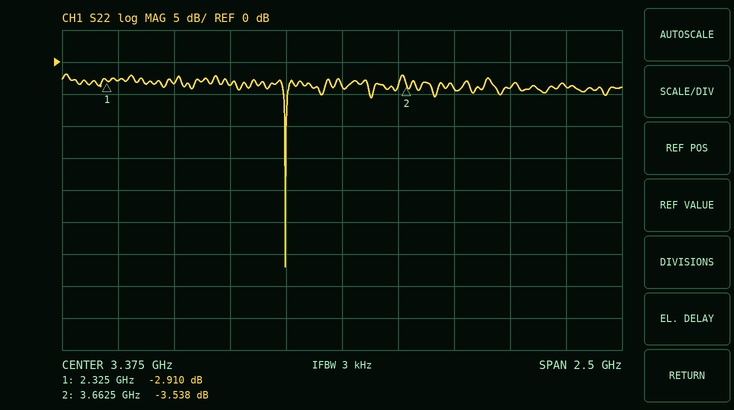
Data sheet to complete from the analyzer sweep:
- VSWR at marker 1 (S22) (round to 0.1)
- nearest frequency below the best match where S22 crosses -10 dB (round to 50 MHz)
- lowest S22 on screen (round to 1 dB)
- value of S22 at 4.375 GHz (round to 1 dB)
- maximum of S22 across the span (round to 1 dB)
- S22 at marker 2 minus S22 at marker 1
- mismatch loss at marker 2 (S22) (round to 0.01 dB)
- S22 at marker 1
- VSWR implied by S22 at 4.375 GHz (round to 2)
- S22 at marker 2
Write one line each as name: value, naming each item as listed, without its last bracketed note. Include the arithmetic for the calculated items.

VSWR at marker 1 (S22): (1 + 0.7153)/(1 − 0.7153) ≈ 6.0
nearest frequency below the best match where S22 crosses -10 dB: 3.10 GHz
lowest S22 on screen: -32 dB
value of S22 at 4.375 GHz: -4 dB
maximum of S22 across the span: -2 dB
S22 at marker 2 minus S22 at marker 1: -3.538 − (-2.91) = -0.628 dB
mismatch loss at marker 2 (S22): −10 log10(1 − 10^(-3.538/10)) ≈ 2.54 dB
S22 at marker 1: -2.910 dB
VSWR implied by S22 at 4.375 GHz: |Γ| = 10^(-4/20) = 0.6310; VSWR = (1 + 0.6310)/(1 − 0.6310) ≈ 4
S22 at marker 2: -3.538 dB
